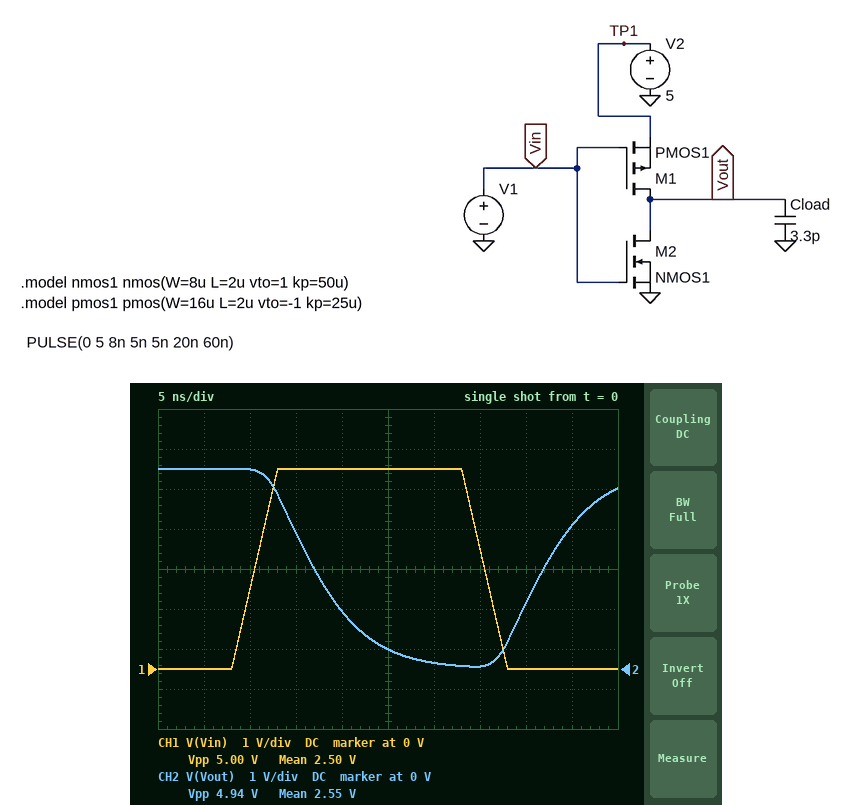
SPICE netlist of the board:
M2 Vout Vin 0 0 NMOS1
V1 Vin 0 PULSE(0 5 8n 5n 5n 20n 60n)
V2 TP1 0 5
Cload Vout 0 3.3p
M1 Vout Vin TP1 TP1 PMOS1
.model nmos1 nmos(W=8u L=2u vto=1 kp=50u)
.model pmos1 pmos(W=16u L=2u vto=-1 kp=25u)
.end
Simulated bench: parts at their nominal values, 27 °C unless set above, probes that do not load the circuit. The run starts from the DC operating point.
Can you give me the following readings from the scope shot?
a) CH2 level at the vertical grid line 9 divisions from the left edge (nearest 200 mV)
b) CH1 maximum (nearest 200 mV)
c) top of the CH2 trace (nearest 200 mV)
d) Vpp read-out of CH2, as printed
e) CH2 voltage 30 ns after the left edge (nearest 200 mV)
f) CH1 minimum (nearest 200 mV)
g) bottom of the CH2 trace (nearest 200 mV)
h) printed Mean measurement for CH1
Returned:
3.6 V
5.0 V
5.0 V
4.94 V
200 mV
0 V
0 V
2.50 V
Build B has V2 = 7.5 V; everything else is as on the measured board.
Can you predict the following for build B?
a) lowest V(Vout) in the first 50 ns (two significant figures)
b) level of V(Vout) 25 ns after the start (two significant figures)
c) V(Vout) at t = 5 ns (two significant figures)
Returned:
650 mV
2.1 V
7.5 V
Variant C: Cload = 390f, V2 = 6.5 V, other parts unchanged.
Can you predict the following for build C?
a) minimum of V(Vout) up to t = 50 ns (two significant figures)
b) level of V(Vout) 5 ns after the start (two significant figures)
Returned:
31 mV
6.5 V
